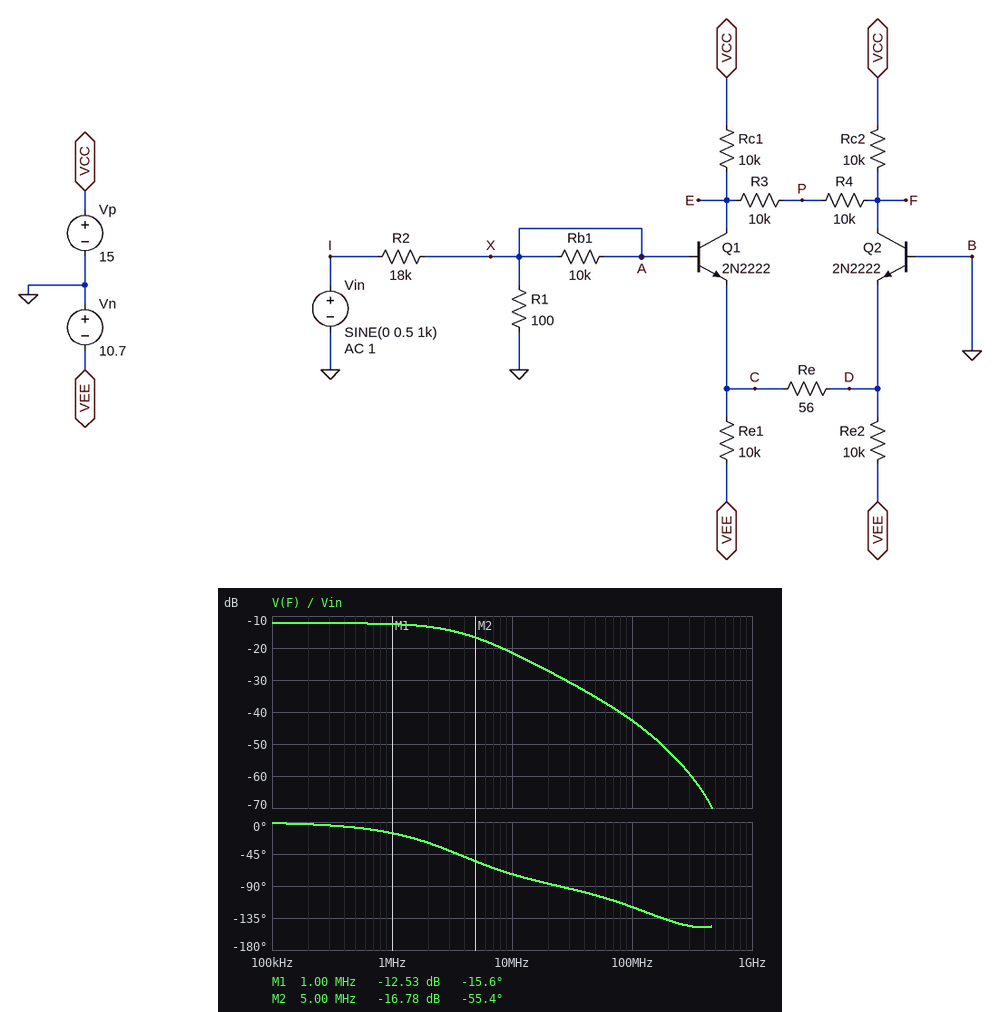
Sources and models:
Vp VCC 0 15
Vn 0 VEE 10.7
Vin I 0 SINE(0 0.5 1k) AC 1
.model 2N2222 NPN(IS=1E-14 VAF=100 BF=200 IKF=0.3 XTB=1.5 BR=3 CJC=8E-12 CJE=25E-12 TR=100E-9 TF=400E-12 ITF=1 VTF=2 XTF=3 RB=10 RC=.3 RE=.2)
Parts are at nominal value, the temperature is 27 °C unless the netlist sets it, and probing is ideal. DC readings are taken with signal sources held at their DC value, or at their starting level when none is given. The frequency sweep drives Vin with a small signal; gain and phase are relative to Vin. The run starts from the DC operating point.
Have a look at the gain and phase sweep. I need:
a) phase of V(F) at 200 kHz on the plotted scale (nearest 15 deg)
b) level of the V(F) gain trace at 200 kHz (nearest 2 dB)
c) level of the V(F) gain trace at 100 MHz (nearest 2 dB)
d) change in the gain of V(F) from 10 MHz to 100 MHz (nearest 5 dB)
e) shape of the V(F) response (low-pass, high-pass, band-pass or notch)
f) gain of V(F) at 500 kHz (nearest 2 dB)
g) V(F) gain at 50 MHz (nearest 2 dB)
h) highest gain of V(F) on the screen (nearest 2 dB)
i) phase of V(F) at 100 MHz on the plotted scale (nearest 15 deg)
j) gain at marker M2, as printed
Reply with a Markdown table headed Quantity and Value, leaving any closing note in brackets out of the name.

| Quantity | Value |
|---|---|
| phase of V(F) at 200 kHz on the plotted scale | 0 deg |
| level of the V(F) gain trace at 200 kHz | -12 dB |
| level of the V(F) gain trace at 100 MHz | -42 dB |
| change in the gain of V(F) from 10 MHz to 100 MHz | -20 dB |
| shape of the V(F) response | low-pass |
| gain of V(F) at 500 kHz | -12 dB |
| V(F) gain at 50 MHz | -36 dB |
| highest gain of V(F) on the screen | -12 dB |
| phase of V(F) at 100 MHz on the plotted scale | -120 deg |
| gain at marker M2, as printed | -16.78 dB |
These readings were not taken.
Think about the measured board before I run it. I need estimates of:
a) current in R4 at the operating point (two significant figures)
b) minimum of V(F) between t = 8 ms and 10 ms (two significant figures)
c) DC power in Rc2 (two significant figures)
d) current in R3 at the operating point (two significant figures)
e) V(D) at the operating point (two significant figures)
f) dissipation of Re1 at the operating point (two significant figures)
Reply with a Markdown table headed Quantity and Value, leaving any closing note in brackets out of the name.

| Quantity | Value |
|---|---|
| current in R4 at the operating point | 2.1 µA |
| minimum of V(F) between t = 8 ms and 10 ms | 4.9 V |
| DC power in Rc2 | 10 mW |
| current in R3 at the operating point | 2.1 µA |
| V(D) at the operating point | -650 mV |
| dissipation of Re1 at the operating point | 10 mW |
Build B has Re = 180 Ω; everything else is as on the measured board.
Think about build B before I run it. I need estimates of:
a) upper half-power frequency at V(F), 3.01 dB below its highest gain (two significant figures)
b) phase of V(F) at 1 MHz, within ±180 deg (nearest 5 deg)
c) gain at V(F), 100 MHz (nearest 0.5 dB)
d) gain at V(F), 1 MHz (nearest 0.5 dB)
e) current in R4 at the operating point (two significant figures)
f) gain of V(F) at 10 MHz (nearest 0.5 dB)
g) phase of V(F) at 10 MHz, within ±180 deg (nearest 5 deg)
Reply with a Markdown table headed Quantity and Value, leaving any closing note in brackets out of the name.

| Quantity | Value |
|---|---|
| upper half-power frequency at V(F), 3.01 dB below its highest gain | 5.1 MHz |
| phase of V(F) at 1 MHz, within ±180 deg | -10 deg |
| gain at V(F), 100 MHz | -46.5 dB |
| gain at V(F), 1 MHz | -19.0 dB |
| current in R4 at the operating point | 1.0 µA |
| gain of V(F) at 10 MHz | -25.5 dB |
| phase of V(F) at 10 MHz, within ±180 deg | -65 deg |
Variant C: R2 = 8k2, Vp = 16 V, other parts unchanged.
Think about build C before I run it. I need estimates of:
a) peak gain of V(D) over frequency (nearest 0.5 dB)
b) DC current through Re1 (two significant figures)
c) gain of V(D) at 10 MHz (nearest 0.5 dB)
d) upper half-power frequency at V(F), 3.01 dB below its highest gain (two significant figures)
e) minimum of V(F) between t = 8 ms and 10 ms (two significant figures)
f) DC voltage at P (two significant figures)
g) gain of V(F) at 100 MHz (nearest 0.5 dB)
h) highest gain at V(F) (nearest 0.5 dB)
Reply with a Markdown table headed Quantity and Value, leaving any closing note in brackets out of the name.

| Quantity | Value |
|---|---|
| peak gain of V(D) over frequency | -50.5 dB |
| DC current through Re1 | 1.0 mA |
| gain of V(D) at 10 MHz | -54.0 dB |
| upper half-power frequency at V(F), 3.01 dB below its highest gain | 3.9 MHz |
| minimum of V(F) between t = 8 ms and 10 ms | 5.7 V |
| DC voltage at P | 6.0 V |
| gain of V(F) at 100 MHz | -35.5 dB |
| highest gain at V(F) | -5.5 dB |
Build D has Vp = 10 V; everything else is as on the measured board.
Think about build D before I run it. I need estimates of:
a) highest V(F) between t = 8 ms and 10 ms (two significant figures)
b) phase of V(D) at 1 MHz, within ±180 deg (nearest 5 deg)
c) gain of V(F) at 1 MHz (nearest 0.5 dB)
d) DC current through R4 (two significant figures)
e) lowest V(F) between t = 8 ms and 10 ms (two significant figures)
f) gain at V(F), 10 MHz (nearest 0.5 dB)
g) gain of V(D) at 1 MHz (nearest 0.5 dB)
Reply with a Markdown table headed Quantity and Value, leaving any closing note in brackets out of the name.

| Quantity | Value |
|---|---|
| highest V(F) between t = 8 ms and 10 ms | 110 mV |
| phase of V(D) at 1 MHz, within ±180 deg | -10 deg |
| gain of V(F) at 1 MHz | -13.5 dB |
| DC current through R4 | 2.2 µA |
| lowest V(F) between t = 8 ms and 10 ms | -140 mV |
| gain at V(F), 10 MHz | -27.0 dB |
| gain of V(D) at 1 MHz | -58.0 dB |
